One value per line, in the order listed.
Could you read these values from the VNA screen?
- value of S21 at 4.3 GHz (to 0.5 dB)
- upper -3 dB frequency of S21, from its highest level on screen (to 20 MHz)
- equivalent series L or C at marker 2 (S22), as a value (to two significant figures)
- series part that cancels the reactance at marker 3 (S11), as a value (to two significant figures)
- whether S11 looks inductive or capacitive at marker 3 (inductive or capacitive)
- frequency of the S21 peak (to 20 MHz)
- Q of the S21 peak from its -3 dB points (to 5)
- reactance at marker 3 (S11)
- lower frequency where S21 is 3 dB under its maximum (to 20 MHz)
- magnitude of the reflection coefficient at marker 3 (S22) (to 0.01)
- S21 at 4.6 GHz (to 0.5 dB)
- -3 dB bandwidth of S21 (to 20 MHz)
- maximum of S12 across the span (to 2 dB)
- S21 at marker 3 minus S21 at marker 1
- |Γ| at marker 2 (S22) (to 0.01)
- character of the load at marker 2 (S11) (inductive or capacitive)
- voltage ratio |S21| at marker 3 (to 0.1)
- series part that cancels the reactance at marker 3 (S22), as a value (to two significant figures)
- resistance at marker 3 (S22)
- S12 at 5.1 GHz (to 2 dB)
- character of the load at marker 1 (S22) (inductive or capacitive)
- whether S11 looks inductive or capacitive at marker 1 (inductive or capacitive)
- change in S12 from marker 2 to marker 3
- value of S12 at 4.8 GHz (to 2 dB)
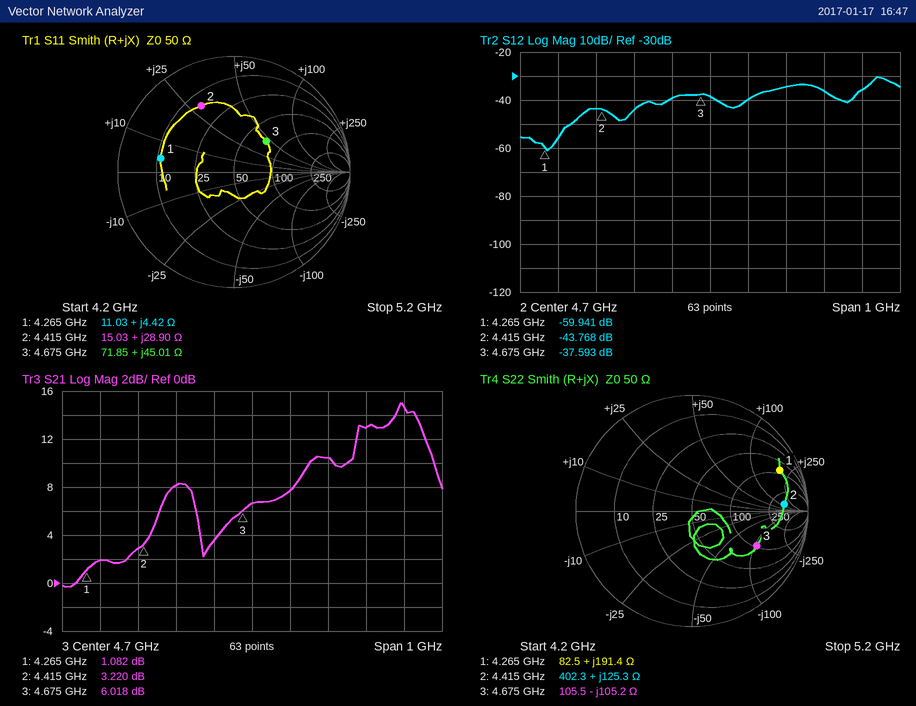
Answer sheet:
2.0 dB
5.16 GHz
4.5 nH
760 fF
inductive
5.10 GHz
30
+45.01 Ω
4.98 GHz
0.63
3.5 dB
180 MHz
-30 dB
4.936 dB
0.80
inductive
2.0
3.6 nH
105.5 Ω
-36 dB
inductive
inductive
6.175 dB
-40 dB
